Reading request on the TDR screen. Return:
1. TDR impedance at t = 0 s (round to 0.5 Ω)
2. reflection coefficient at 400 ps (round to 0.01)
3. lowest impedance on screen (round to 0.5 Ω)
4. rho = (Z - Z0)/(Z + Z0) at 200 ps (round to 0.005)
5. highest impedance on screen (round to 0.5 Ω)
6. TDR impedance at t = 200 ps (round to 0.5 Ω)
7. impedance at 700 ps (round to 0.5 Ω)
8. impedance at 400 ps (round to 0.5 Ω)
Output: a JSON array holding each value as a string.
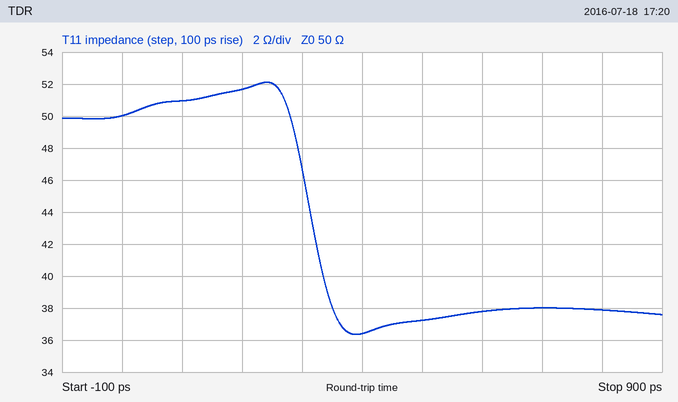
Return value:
["50.0 Ω", "-0.16", "36.5 Ω", "+0.015", "52.0 Ω", "51.5 Ω", "38.0 Ω", "36.5 Ω"]
